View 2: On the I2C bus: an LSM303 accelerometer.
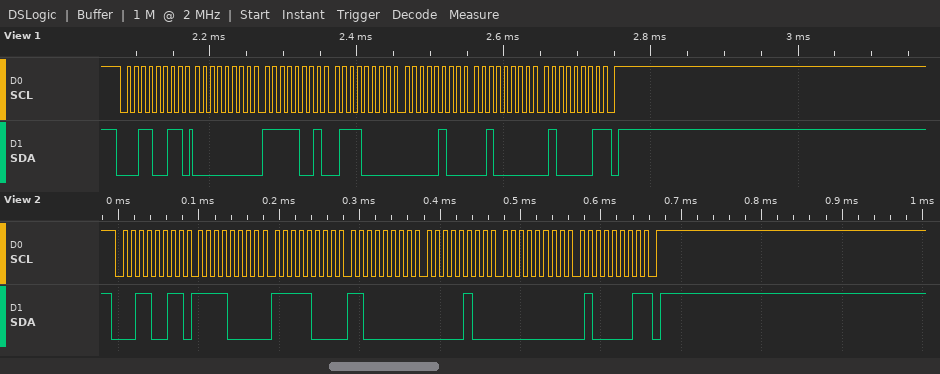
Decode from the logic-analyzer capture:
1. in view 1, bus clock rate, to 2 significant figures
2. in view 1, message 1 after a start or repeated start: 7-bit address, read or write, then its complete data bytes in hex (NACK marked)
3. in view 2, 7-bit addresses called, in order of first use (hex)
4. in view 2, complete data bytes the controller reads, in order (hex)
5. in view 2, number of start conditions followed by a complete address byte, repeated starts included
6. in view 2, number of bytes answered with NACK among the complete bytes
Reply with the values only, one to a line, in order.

100 kHz
0x19 read: 00 F9 70 04 20 41 NACK
0x19
F0 F8 C0 04 00 41
1
1
